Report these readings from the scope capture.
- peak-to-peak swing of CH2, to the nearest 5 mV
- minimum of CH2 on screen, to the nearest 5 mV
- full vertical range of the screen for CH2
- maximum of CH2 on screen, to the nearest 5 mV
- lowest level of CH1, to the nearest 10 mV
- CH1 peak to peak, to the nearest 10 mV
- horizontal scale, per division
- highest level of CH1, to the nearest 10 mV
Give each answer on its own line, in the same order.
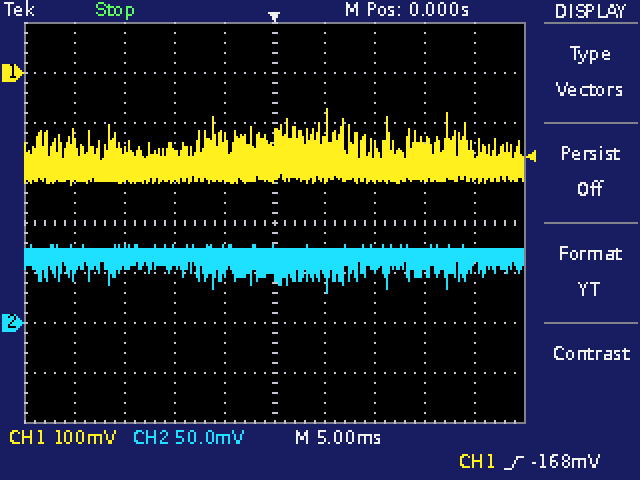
50 mV
30 mV
400 mV
80 mV
-220 mV
150 mV
5 ms
-70 mV
